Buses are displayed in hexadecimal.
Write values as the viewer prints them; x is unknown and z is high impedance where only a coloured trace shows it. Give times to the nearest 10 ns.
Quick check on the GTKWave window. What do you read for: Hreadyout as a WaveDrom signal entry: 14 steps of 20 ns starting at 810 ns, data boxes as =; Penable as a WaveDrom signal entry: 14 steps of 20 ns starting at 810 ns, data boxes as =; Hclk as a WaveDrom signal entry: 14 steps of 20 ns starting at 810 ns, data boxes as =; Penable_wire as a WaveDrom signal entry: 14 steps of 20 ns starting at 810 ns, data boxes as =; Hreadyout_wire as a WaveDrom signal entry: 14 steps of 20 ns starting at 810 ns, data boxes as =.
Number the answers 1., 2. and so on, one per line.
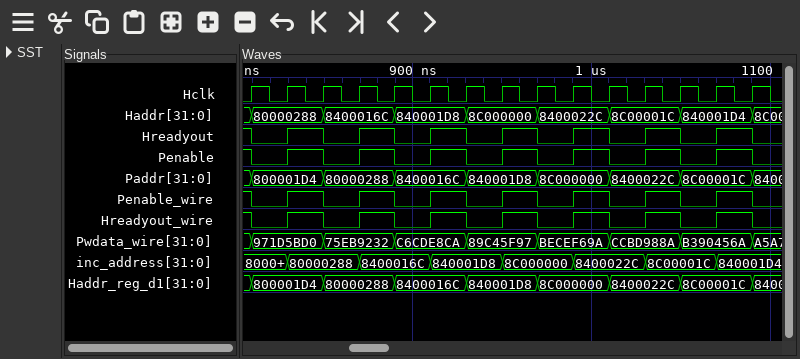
1. {name: 'Hreadyout', wave: '01010101010101'}
2. {name: 'Penable', wave: '01010101010101'}
3. {name: 'Hclk', wave: 'p.............'}
4. {name: 'Penable_wire', wave: '01010101010101'}
5. {name: 'Hreadyout_wire', wave: '01010101010101'}
